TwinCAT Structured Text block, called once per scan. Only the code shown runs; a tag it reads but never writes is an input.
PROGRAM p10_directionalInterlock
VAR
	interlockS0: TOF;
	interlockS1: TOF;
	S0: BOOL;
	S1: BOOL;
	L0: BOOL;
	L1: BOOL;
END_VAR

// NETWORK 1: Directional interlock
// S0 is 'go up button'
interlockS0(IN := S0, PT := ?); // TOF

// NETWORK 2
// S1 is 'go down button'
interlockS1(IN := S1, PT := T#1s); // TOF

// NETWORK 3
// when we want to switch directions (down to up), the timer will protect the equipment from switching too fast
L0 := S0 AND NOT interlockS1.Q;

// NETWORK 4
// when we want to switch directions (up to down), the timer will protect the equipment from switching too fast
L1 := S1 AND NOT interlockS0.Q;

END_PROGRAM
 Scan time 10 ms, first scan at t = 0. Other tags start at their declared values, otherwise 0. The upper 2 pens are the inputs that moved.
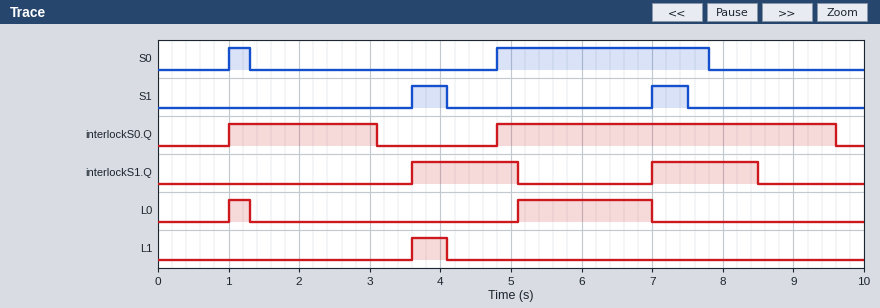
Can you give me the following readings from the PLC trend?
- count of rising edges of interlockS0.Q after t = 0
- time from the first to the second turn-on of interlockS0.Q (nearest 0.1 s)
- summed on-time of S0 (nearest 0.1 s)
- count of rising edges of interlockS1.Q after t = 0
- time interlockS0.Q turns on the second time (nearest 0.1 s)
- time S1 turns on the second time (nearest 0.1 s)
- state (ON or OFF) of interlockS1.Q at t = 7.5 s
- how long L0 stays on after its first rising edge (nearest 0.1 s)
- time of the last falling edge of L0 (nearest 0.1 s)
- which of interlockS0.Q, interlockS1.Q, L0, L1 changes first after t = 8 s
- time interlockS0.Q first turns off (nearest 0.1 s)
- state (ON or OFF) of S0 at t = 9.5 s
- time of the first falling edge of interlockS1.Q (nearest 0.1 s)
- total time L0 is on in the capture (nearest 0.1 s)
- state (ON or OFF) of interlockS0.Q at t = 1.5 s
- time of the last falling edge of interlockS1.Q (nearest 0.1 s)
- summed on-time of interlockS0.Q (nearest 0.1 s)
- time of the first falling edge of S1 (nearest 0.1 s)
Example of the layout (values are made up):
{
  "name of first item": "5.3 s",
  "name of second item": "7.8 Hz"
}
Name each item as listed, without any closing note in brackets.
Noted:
{
  "count of rising edges of interlockS0.Q after t = 0": "2",
  "time from the first to the second turn-on of interlockS0.Q": "3.8 s",
  "summed on-time of S0": "3.3 s",
  "count of rising edges of interlockS1.Q after t = 0": "2",
  "time interlockS0.Q turns on the second time": "4.8 s",
  "time S1 turns on the second time": "7.0 s",
  "state (ON or OFF) of interlockS1.Q at t = 7.5 s": "ON",
  "how long L0 stays on after its first rising edge": "0.3 s",
  "time of the last falling edge of L0": "7.0 s",
  "which of interlockS0.Q, interlockS1.Q, L0, L1 changes first after t = 8 s": "interlockS1.Q",
  "time interlockS0.Q first turns off": "3.1 s",
  "state (ON or OFF) of S0 at t = 9.5 s": "OFF",
  "time of the first falling edge of interlockS1.Q": "5.1 s",
  "total time L0 is on in the capture": "2.2 s",
  "state (ON or OFF) of interlockS0.Q at t = 1.5 s": "ON",
  "time of the last falling edge of interlockS1.Q": "8.5 s",
  "summed on-time of interlockS0.Q": "6.9 s",
  "time of the first falling edge of S1": "4.1 s"
}
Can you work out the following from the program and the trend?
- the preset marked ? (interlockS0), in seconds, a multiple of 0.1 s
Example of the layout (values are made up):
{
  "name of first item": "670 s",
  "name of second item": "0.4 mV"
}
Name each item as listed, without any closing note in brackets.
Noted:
{
  "the preset marked ? (interlockS0), in seconds, a multiple of 0.1 s": "1.8 s"
}
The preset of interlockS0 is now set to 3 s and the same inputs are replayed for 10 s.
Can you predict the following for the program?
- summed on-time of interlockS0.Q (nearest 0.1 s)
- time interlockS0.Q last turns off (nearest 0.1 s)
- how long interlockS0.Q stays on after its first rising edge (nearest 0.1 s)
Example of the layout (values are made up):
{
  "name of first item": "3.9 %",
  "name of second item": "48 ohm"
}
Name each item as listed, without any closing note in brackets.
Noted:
{
  "summed on-time of interlockS0.Q": "8.5 s",
  "time interlockS0.Q last turns off": "4.3 s",
  "how long interlockS0.Q stays on after its first rising edge": "3.3 s"
}
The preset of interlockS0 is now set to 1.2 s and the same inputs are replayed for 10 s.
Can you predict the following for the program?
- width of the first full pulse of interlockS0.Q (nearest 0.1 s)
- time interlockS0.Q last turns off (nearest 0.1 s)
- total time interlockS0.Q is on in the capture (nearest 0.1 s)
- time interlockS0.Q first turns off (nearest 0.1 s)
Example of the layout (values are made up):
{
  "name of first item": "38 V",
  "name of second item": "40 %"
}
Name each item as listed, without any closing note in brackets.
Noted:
{
  "width of the first full pulse of interlockS0.Q": "1.5 s",
  "time interlockS0.Q last turns off": "9.0 s",
  "total time interlockS0.Q is on in the capture": "5.7 s",
  "time interlockS0.Q first turns off": "2.5 s"
}
